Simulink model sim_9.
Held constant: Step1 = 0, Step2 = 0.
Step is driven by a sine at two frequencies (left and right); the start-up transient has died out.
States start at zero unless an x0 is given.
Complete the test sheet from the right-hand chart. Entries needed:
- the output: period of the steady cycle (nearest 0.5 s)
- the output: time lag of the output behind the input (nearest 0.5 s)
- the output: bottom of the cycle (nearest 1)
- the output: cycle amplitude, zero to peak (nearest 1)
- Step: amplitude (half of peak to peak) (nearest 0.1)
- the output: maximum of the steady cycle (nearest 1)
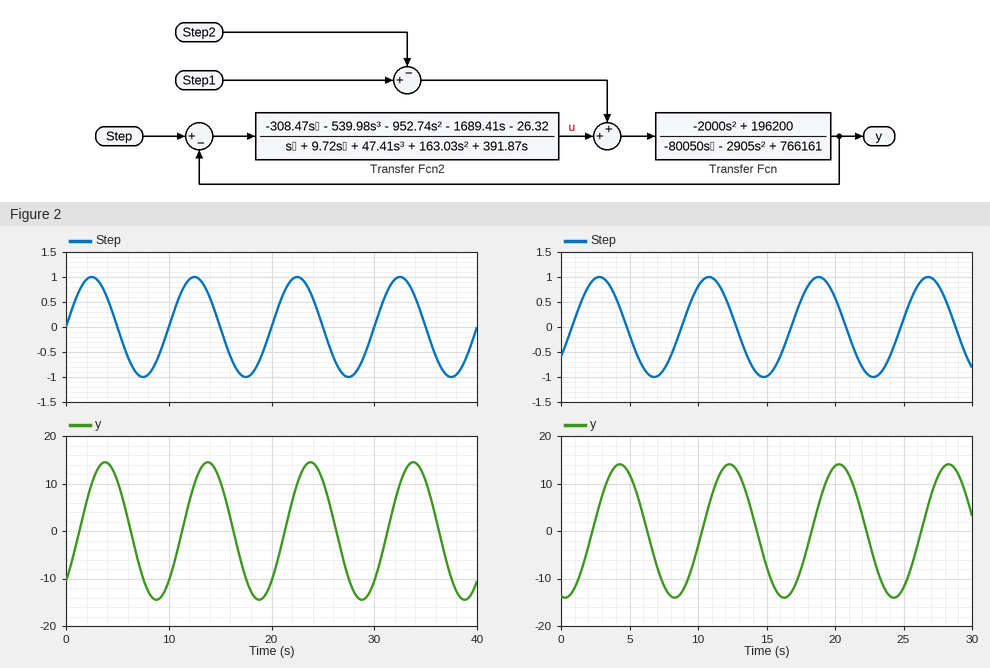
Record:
8.0 s
1.5 s
-14
14
1.0
14
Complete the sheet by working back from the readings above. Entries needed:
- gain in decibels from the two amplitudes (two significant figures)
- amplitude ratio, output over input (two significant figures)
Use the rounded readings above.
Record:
23 dB
14
